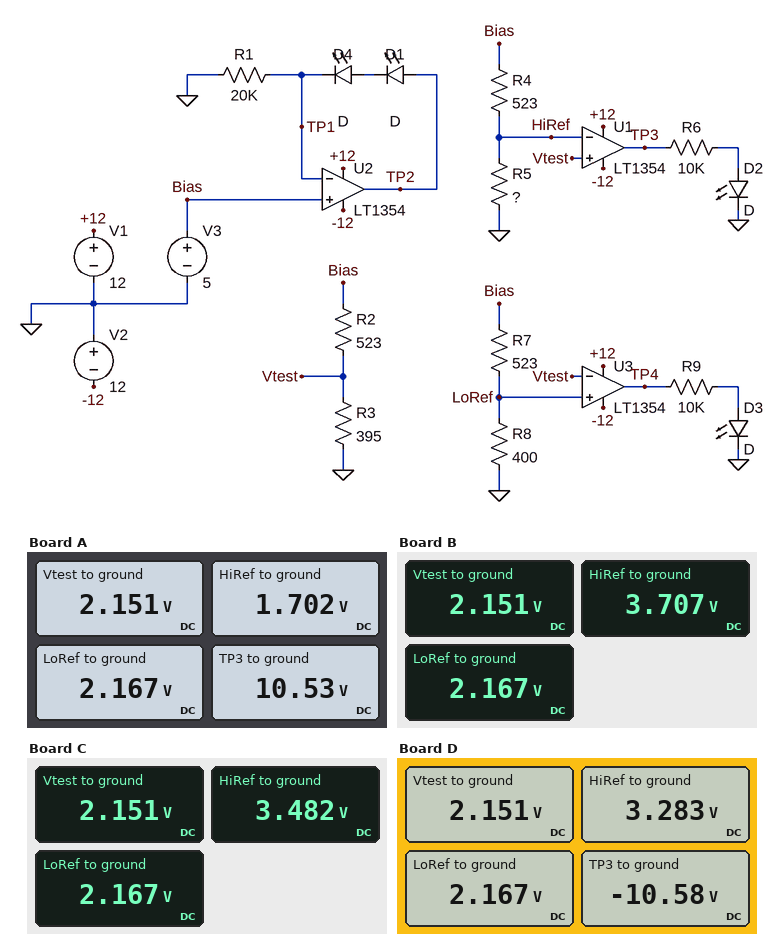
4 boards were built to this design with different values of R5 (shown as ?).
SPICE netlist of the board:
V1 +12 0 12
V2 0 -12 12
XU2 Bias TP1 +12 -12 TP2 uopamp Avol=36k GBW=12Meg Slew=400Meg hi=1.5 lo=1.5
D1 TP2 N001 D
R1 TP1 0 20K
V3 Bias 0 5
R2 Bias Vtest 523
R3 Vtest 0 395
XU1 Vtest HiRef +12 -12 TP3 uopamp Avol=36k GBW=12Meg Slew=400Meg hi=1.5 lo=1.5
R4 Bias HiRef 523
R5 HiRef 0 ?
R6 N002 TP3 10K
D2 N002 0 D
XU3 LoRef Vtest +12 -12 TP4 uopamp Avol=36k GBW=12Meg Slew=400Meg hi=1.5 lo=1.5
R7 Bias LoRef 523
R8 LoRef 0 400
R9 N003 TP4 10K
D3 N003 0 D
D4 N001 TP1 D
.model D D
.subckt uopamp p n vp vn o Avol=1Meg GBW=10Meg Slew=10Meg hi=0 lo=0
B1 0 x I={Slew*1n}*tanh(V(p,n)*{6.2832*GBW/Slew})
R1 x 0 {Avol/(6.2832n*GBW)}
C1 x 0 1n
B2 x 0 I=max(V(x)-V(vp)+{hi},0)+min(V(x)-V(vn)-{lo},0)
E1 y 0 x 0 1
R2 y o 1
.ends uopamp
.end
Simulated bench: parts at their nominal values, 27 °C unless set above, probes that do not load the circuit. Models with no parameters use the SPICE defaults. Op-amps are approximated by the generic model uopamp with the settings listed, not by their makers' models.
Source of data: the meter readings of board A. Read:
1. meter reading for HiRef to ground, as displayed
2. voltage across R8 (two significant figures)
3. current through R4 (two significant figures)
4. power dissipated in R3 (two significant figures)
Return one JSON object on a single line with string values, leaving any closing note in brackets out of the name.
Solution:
{"meter reading for HiRef to ground, as displayed": "1.702 V", "voltage across R8": "2.2 V", "current through R4": "6.3 mA", "power dissipated in R3": "12 mW"}
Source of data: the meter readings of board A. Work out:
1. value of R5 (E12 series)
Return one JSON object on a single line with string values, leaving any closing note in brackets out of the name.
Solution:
{"value of R5": "270 Ω"}
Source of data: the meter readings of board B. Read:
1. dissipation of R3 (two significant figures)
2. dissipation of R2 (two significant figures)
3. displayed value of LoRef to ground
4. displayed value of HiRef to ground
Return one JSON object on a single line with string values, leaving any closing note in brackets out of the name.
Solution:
{"dissipation of R3": "12 mW", "dissipation of R2": "16 mW", "displayed value of LoRef to ground": "2.167 V", "displayed value of HiRef to ground": "3.707 V"}
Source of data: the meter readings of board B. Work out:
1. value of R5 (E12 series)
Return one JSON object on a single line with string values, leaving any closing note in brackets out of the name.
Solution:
{"value of R5": "1.5 kΩ"}
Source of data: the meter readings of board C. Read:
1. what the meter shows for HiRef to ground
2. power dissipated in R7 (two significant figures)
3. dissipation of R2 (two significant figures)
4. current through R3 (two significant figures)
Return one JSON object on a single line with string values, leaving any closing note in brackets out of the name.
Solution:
{"what the meter shows for HiRef to ground": "3.482 V", "power dissipated in R7": "15 mW", "dissipation of R2": "16 mW", "current through R3": "5.4 mA"}
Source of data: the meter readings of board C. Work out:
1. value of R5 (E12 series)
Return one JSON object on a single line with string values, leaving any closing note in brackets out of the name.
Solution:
{"value of R5": "1.2 kΩ"}
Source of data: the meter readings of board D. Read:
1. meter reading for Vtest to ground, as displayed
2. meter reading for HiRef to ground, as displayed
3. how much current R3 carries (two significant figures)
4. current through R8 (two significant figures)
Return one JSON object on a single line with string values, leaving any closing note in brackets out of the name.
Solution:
{"meter reading for Vtest to ground, as displayed": "2.151 V", "meter reading for HiRef to ground, as displayed": "3.283 V", "how much current R3 carries": "5.4 mA", "current through R8": "5.4 mA"}
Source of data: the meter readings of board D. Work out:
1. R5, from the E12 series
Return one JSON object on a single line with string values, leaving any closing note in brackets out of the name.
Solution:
{"R5, from the E12 series": "1 kΩ"}
